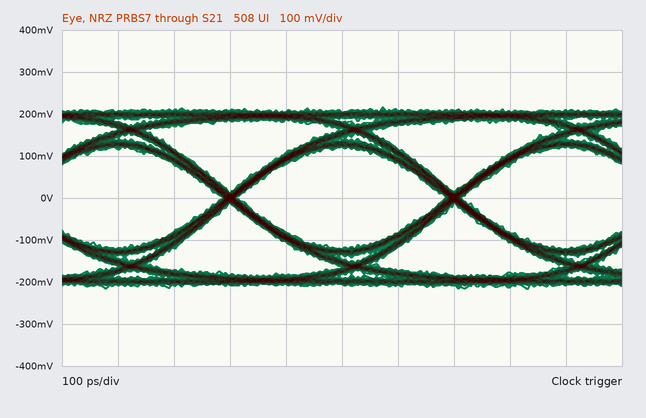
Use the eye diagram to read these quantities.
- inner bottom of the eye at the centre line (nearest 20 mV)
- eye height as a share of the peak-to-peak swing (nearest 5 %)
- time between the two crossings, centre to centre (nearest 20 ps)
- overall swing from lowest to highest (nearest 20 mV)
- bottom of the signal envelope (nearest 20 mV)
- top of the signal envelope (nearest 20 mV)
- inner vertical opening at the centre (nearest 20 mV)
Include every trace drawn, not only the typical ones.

-120 mV
55 %
400 ps
440 mV
-220 mV
220 mV
240 mV
